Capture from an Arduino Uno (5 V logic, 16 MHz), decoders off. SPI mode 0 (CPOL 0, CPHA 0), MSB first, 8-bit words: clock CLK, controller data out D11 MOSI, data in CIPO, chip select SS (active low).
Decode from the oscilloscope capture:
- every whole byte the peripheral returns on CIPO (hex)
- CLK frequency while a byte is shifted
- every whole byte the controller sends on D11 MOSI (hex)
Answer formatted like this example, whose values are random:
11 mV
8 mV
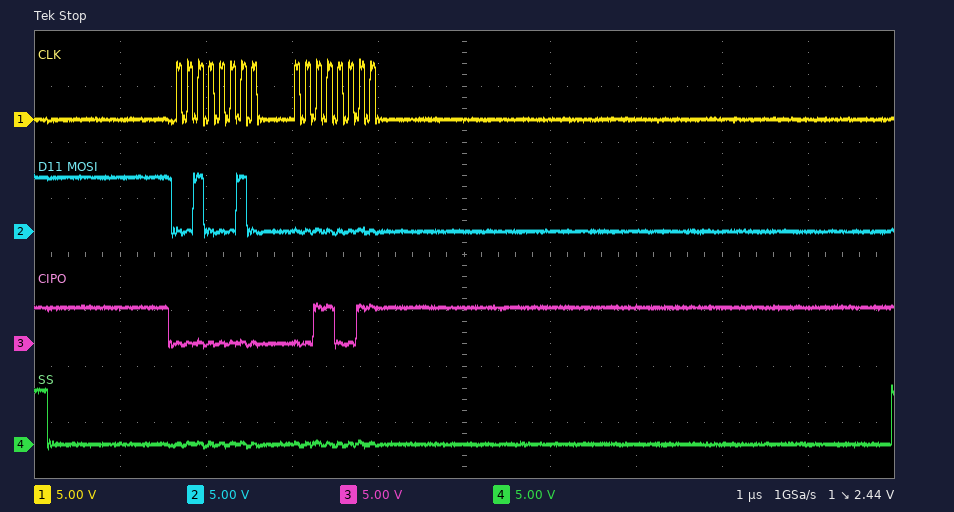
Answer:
00 33
8 MHz
22 00
